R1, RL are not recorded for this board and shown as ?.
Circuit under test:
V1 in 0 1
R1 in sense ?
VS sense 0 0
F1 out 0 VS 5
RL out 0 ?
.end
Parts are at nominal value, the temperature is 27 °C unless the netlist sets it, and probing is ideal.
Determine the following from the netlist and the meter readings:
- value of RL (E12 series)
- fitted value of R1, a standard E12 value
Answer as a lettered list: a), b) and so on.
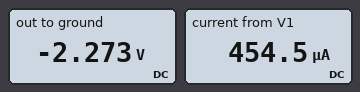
a) 1 kΩ
b) 2.2 kΩ
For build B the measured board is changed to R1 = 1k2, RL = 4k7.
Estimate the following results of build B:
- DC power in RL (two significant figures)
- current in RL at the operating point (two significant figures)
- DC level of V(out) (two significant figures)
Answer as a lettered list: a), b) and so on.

a) 82 mW
b) 4.2 mA
c) -20 V
